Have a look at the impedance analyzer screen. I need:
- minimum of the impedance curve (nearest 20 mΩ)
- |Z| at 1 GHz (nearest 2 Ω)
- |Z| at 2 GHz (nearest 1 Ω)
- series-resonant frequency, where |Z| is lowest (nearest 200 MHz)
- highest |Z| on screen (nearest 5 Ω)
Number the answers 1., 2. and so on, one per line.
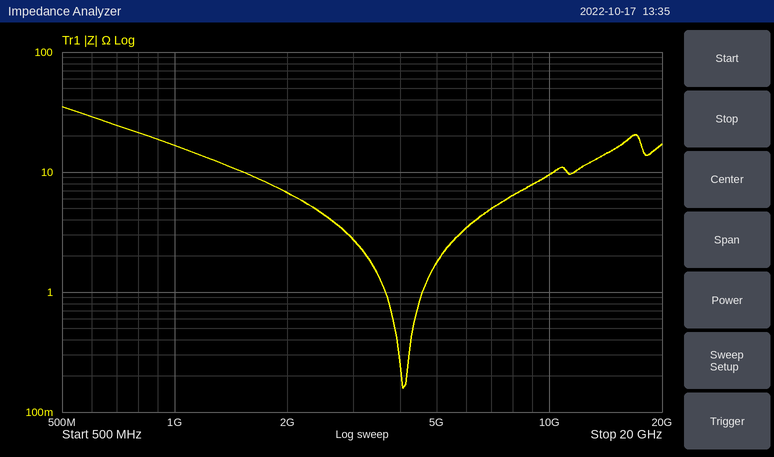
1. 160 mΩ
2. 16 Ω
3. 7 Ω
4. 4.0 GHz
5. 35 Ω
